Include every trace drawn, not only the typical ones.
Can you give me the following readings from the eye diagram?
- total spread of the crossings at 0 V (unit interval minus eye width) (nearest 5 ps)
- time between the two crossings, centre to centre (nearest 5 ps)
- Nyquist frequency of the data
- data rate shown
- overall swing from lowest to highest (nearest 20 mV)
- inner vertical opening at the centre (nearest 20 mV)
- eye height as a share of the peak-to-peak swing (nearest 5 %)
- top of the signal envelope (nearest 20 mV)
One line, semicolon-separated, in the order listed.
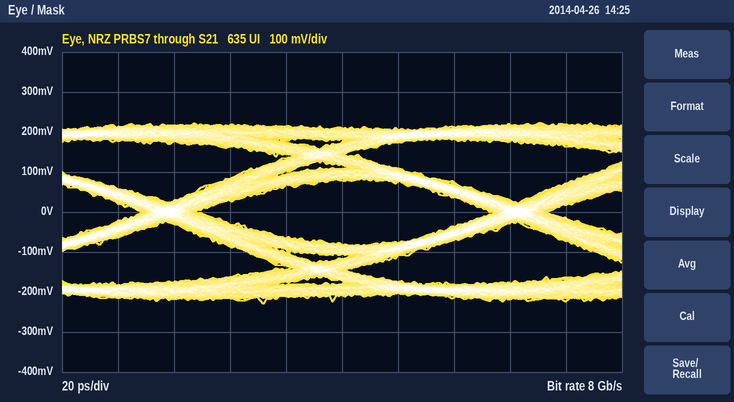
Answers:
20 ps; 125 ps; 4 GHz; 8 Gb/s; 460 mV; 160 mV; 35 %; 220 mV
